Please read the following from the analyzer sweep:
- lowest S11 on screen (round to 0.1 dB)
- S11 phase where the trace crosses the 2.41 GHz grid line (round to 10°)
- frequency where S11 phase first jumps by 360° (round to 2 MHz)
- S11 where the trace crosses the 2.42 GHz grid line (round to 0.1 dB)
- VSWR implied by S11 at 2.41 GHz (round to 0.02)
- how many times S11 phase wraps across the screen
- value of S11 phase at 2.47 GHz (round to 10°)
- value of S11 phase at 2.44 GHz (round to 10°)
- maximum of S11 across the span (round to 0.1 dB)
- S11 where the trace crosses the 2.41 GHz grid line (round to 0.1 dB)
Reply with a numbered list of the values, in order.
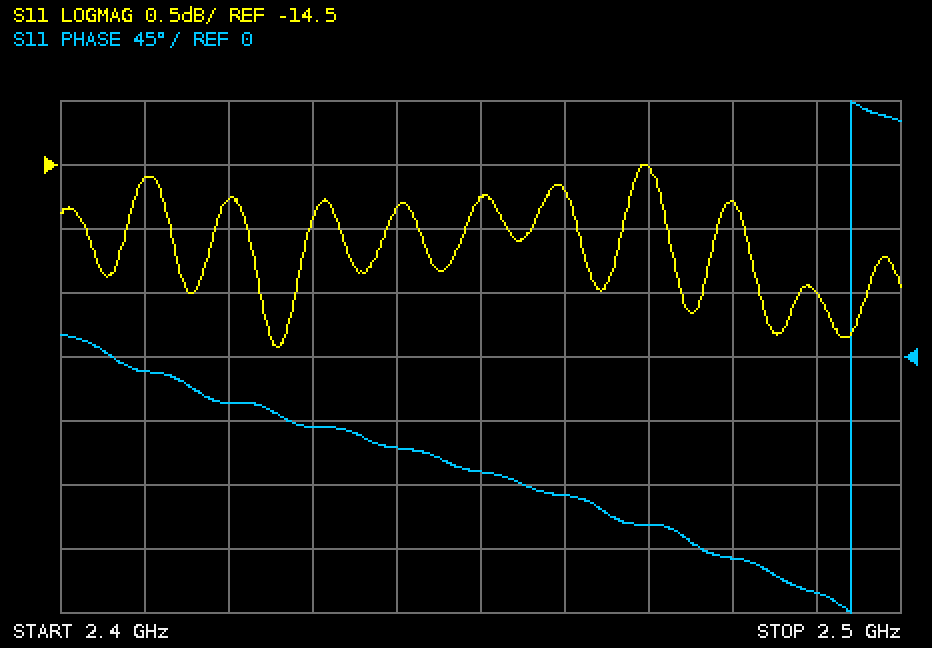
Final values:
1. -15.9 dB
2. -10°
3. 2.494 GHz
4. -14.8 dB
5. 1.46
6. 1
7. -120°
8. -60°
9. -14.5 dB
10. -14.6 dB
